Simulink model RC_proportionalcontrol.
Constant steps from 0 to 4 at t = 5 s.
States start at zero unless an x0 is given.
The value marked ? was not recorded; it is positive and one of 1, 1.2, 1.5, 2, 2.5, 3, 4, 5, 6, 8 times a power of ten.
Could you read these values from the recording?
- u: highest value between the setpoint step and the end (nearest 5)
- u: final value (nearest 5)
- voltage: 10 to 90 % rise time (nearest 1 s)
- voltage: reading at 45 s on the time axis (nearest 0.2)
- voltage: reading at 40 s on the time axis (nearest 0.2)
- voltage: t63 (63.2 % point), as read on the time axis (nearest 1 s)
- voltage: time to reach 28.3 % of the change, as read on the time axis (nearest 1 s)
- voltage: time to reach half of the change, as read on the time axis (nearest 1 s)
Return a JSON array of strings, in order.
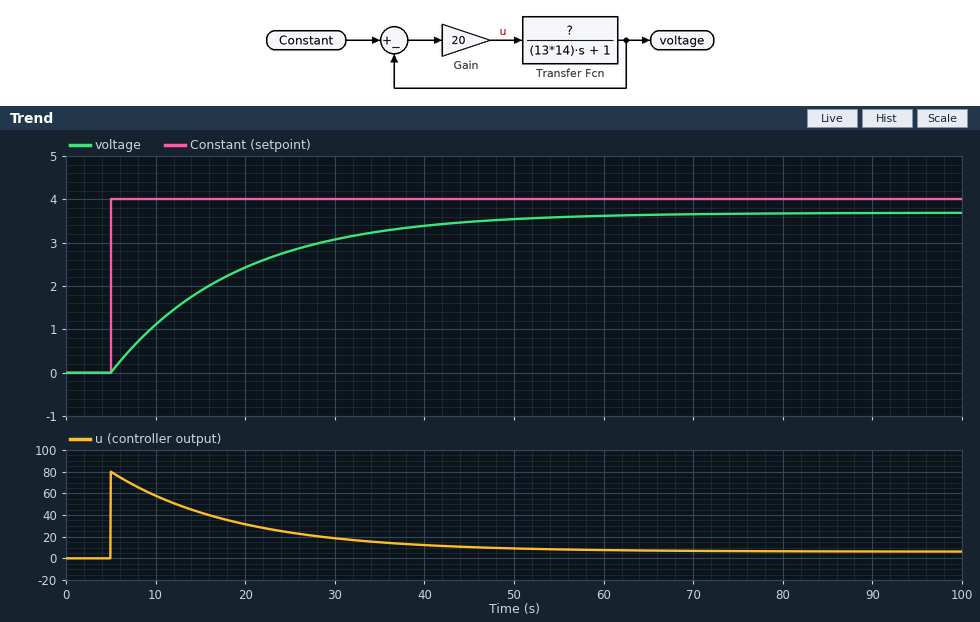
["80", "5", "31 s", "3.4", "3.4", "19 s", "10 s", "15 s"]
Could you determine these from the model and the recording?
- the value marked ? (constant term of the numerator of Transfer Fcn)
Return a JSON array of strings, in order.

["0.6"]
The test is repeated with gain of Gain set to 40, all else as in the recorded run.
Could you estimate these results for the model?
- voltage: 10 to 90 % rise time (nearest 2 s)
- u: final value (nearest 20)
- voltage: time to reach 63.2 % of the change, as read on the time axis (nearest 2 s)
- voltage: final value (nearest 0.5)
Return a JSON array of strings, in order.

["16 s", "0", "12 s", "4.0"]
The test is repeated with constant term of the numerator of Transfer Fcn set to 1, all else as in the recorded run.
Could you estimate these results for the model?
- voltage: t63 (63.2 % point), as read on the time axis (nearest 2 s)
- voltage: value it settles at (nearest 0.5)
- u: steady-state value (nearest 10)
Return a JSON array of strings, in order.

["14 s", "4.0", "0"]
